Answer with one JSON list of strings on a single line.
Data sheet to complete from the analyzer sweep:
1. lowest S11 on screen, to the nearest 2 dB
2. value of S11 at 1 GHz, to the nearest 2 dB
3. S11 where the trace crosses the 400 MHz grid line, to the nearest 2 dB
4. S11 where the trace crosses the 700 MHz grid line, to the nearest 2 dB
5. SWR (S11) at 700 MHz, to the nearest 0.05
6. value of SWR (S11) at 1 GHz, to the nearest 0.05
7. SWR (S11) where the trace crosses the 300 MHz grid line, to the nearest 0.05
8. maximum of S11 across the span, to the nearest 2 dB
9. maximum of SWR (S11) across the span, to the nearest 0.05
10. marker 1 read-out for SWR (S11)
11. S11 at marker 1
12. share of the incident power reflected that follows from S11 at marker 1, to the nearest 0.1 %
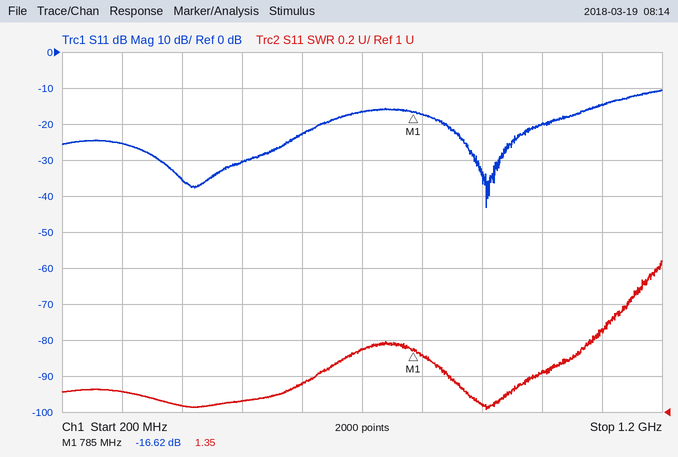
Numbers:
["-44 dB", "-20 dB", "-36 dB", "-16 dB", "1.35", "1.20", "1.10", "-10 dB", "1.85", "1.35", "-16.62 dB", "2.2 %"]
